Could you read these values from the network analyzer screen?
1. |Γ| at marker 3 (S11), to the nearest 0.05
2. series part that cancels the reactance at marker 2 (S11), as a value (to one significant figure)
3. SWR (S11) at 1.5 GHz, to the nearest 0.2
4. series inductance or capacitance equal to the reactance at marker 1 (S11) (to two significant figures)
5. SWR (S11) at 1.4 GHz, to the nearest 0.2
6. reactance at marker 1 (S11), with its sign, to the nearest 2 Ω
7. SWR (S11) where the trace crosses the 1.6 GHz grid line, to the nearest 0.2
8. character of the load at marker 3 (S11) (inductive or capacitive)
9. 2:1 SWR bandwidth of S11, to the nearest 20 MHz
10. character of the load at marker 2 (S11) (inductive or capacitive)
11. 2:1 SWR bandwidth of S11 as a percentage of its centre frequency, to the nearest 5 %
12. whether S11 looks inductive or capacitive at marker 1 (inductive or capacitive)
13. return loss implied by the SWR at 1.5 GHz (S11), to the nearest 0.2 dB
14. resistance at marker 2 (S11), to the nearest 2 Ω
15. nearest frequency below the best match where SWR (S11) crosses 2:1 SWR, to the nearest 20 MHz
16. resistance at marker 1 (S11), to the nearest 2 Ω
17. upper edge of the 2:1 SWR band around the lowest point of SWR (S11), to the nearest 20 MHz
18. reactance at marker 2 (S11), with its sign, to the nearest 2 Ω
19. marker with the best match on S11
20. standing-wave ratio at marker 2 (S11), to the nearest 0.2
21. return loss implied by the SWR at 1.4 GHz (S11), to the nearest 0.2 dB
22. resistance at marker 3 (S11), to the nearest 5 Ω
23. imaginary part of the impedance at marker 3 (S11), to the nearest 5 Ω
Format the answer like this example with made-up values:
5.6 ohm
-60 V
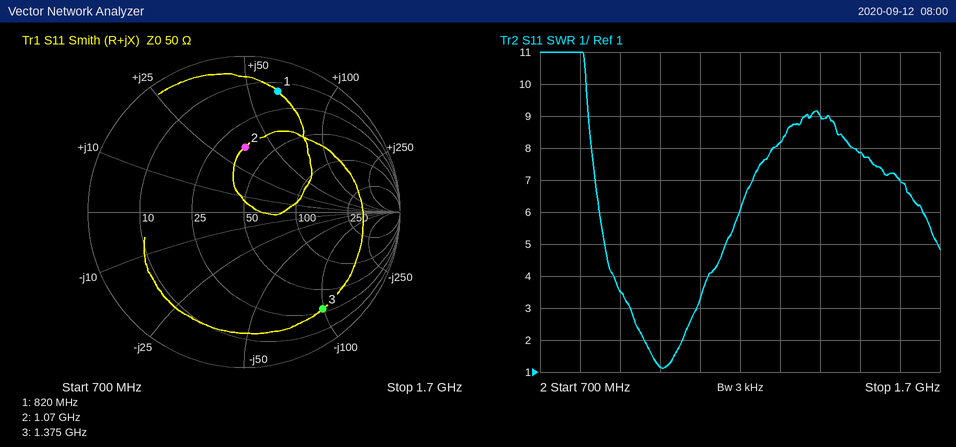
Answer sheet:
0.80
4 pF
7.8
12 nH
9.0
+64 Ω
7.0
capacitive
100 MHz
inductive
10 %
inductive
2.2 dB
36 Ω
960 MHz
14 Ω
1.06 GHz
+36 Ω
marker 2
2.4
2.0 dB
30 Ω
-100 Ω
